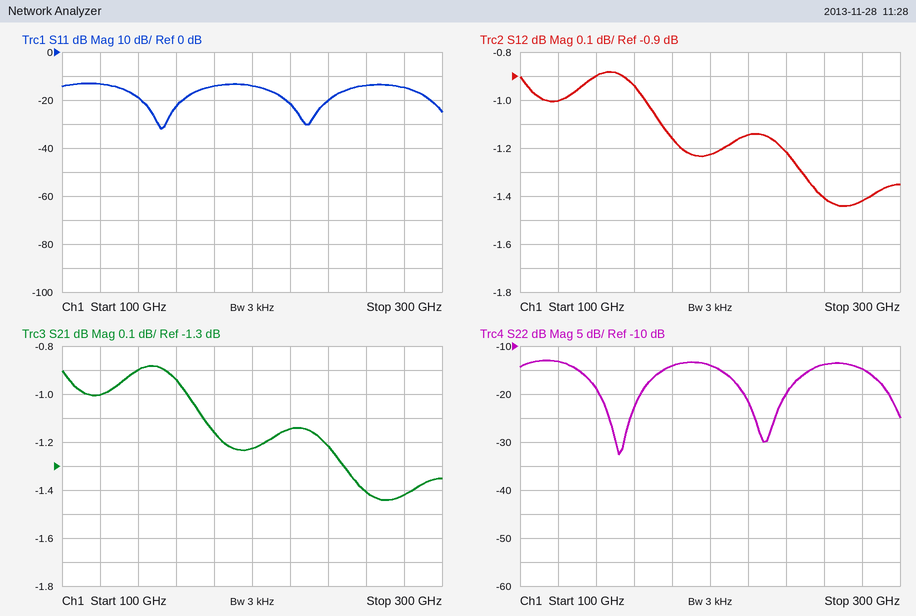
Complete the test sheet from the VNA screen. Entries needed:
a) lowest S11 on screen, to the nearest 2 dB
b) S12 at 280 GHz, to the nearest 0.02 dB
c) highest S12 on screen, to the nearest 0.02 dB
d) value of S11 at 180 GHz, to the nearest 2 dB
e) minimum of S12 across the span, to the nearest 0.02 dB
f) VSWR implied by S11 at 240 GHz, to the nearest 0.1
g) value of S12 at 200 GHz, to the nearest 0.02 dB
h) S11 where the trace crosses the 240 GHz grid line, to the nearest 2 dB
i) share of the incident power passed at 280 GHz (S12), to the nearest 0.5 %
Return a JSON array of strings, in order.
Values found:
["-32 dB", "-1.42 dB", "-0.88 dB", "-14 dB", "-1.44 dB", "1.2", "-1.22 dB", "-20 dB", "72.0 %"]
